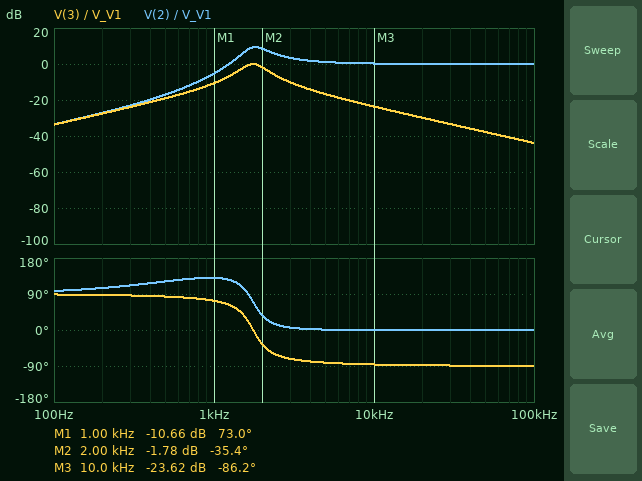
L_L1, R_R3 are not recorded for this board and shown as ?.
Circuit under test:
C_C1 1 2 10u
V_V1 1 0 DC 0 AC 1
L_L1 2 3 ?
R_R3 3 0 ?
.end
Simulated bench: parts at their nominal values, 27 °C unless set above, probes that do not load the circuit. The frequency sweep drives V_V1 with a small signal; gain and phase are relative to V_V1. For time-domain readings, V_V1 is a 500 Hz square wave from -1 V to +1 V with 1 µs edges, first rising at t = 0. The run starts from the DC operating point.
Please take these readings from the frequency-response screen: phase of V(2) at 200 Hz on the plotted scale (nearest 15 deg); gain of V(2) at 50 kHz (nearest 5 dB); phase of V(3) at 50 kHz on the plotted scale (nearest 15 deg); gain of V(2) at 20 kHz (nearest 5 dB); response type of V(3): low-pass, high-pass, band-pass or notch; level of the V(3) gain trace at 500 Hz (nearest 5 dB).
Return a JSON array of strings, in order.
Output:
["105 deg", "0 dB", "-90 deg", "0 dB", "band-pass", "-20 dB"]
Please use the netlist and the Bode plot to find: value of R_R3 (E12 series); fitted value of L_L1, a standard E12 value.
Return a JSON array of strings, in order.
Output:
["3.3 Ω", "820 µH"]
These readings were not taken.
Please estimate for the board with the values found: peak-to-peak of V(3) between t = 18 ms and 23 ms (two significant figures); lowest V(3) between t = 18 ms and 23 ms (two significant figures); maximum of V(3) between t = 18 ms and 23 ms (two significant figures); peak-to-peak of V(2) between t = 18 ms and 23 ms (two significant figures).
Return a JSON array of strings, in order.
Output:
["1.2 V", "-580 mV", "580 mV", "4.1 V"]
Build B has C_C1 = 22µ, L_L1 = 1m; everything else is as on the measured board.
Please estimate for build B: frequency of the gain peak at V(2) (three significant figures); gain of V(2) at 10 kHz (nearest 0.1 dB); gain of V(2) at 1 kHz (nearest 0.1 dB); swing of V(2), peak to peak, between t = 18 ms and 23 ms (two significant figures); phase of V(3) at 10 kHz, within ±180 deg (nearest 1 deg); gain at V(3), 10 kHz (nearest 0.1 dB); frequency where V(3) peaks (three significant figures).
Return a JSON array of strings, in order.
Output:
["1.13 kHz", "0.1 dB", "6.3 dB", "3.3 V", "-87 deg", "-25.5 dB", "1.07 kHz"]
